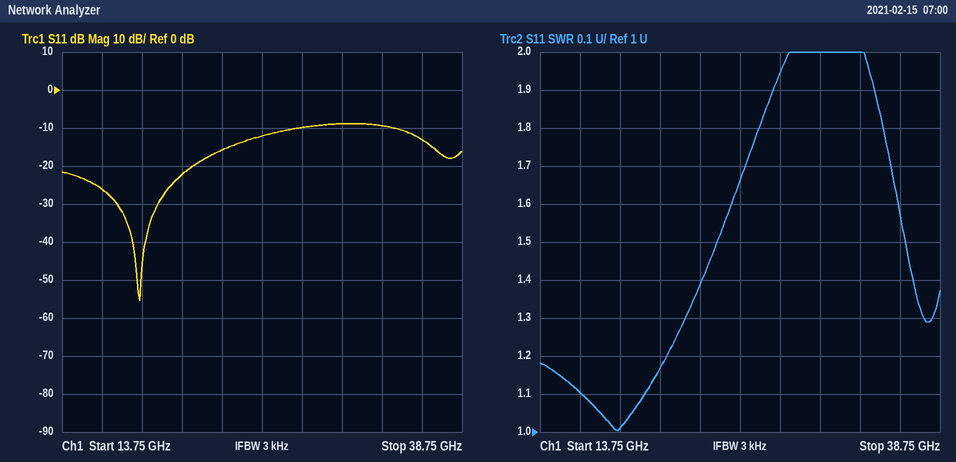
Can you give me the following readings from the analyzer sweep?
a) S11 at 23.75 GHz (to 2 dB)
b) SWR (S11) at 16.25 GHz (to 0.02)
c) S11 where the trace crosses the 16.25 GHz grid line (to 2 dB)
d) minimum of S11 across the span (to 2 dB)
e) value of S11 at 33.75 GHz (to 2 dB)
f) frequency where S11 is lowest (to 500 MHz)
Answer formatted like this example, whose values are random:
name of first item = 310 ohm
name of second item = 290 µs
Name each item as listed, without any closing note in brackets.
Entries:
S11 at 23.75 GHz = -16 dB
SWR (S11) at 16.25 GHz = 1.10
S11 where the trace crosses the 16.25 GHz grid line = -26 dB
minimum of S11 across the span = -56 dB
value of S11 at 33.75 GHz = -10 dB
frequency where S11 is lowest = 18.5 GHz
